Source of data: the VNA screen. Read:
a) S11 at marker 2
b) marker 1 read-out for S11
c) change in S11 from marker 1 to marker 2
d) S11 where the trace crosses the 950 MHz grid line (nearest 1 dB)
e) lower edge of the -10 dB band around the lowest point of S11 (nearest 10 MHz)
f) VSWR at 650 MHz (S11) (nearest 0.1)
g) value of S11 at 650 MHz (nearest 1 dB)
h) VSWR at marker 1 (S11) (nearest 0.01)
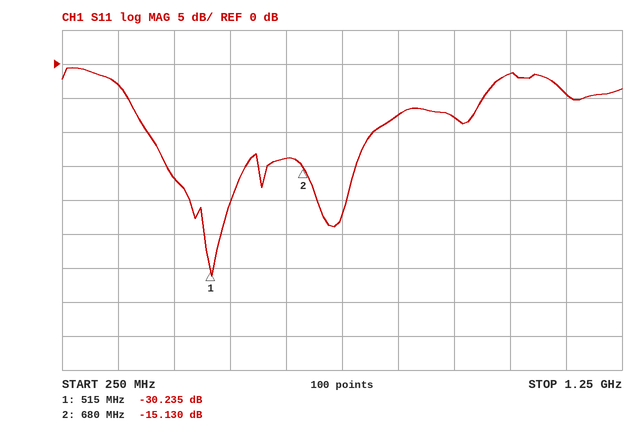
-15.130 dB
-30.235 dB
15.105 dB
-8 dB
400 MHz
1.5
-14 dB
1.06
